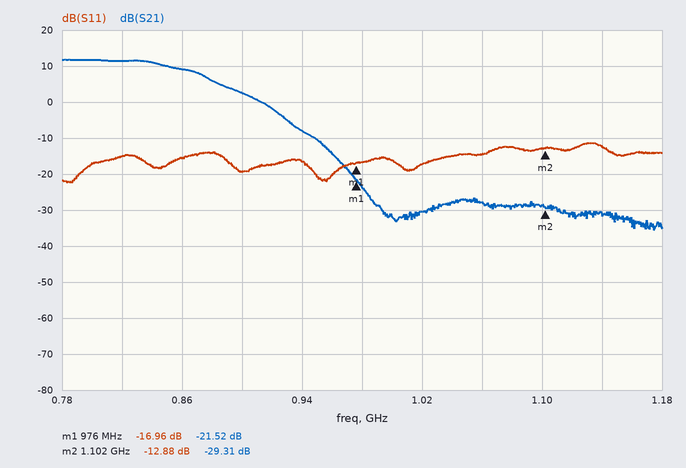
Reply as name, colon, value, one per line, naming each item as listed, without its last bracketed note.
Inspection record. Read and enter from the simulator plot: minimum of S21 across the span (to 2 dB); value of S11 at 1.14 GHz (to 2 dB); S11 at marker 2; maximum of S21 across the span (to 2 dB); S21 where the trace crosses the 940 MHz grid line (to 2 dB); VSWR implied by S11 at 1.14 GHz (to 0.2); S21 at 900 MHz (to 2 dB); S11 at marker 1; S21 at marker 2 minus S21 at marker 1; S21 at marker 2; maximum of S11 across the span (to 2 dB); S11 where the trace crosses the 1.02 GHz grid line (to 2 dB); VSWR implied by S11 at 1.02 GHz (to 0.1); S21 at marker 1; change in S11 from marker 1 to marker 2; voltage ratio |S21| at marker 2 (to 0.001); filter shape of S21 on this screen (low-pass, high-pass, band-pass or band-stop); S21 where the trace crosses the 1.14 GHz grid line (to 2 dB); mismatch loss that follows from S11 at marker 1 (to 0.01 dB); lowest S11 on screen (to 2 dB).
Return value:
minimum of S21 across the span: -36 dB
value of S11 at 1.14 GHz: -12 dB
S11 at marker 2: -12.88 dB
maximum of S21 across the span: 12 dB
S21 where the trace crosses the 940 MHz grid line: -8 dB
VSWR implied by S11 at 1.14 GHz: 1.6
S21 at 900 MHz: 2 dB
S11 at marker 1: -16.96 dB
S21 at marker 2 minus S21 at marker 1: -7.79 dB
S21 at marker 2: -29.31 dB
maximum of S11 across the span: -12 dB
S11 where the trace crosses the 1.02 GHz grid line: -18 dB
VSWR implied by S11 at 1.02 GHz: 1.3
S21 at marker 1: -21.52 dB
change in S11 from marker 1 to marker 2: 4.08 dB
voltage ratio |S21| at marker 2: 0.034
filter shape of S21 on this screen: low-pass
S21 where the trace crosses the 1.14 GHz grid line: -32 dB
mismatch loss that follows from S11 at marker 1: 0.09 dB
lowest S11 on screen: -22 dB
